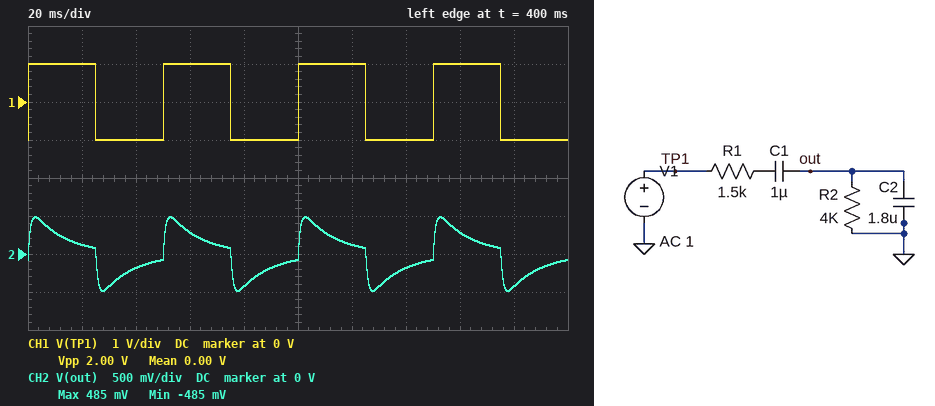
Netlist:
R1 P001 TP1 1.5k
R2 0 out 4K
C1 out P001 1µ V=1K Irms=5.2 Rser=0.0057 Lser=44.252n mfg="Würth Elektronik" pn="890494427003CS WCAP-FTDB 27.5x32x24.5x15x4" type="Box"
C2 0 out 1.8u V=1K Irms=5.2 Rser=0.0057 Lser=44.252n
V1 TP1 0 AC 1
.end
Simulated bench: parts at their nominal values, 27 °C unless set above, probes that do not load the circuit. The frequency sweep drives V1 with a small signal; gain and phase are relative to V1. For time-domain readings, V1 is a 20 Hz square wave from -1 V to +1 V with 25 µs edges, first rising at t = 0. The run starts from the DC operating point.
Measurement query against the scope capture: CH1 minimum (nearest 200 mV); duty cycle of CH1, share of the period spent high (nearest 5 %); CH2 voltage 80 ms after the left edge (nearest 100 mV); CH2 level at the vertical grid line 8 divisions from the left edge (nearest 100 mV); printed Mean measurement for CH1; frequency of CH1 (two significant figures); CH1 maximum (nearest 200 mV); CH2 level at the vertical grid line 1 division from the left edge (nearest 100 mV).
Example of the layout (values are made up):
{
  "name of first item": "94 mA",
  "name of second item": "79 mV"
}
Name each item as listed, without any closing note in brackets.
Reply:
{
  "CH1 minimum": "-1.0 V",
  "duty cycle of CH1, share of the period spent high": "50 %",
  "CH2 voltage 80 ms after the left edge": "-400 mV",
  "CH2 level at the vertical grid line 8 divisions from the left edge": "300 mV",
  "printed Mean measurement for CH1": "0.00 V",
  "frequency of CH1": "20 Hz",
  "CH1 maximum": "1.0 V",
  "CH2 level at the vertical grid line 1 division from the left edge": "100 mV"
}
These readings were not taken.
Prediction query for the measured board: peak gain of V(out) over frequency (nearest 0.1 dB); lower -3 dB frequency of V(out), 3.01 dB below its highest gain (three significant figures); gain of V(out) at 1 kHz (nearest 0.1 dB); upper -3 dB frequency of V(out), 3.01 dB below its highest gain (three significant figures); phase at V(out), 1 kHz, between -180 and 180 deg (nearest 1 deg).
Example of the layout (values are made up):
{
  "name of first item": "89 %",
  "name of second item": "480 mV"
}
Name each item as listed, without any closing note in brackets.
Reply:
{
  "peak gain of V(out) over frequency": "-10.0 dB",
  "lower -3 dB frequency of V(out), 3.01 dB below its highest gain": "11.8 Hz",
  "gain of V(out) at 1 kHz": "-24.7 dB",
  "upper -3 dB frequency of V(out), 3.01 dB below its highest gain": "199 Hz",
  "phase at V(out), 1 kHz, between -180 and 180 deg": "-79 deg"
}
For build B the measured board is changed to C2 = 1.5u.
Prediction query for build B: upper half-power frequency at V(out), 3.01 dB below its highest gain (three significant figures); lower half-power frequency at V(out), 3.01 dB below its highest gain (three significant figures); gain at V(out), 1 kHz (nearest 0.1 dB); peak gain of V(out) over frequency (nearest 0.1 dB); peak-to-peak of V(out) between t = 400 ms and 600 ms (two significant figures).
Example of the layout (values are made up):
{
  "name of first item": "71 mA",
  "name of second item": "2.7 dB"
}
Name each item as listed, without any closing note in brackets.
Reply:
{
  "upper half-power frequency at V(out), 3.01 dB below its highest gain": "216 Hz",
  "lower half-power frequency at V(out), 3.01 dB below its highest gain": "13.0 Hz",
  "gain at V(out), 1 kHz": "-23.2 dB",
  "peak gain of V(out) over frequency": "-9.2 dB",
  "peak-to-peak of V(out) between t = 400 ms and 600 ms": "1.1 V"
}
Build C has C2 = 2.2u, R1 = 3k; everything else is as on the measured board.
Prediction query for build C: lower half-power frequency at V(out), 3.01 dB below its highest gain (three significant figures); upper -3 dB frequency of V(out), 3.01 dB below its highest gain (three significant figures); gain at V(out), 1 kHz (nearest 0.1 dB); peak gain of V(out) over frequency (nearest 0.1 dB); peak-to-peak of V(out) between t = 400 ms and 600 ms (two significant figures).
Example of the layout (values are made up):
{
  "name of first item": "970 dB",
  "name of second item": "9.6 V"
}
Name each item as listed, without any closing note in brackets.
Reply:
{
  "lower half-power frequency at V(out), 3.01 dB below its highest gain": "9.19 Hz",
  "upper -3 dB frequency of V(out), 3.01 dB below its highest gain": "104 Hz",
  "gain at V(out), 1 kHz": "-32.4 dB",
  "peak gain of V(out) over frequency": "-11.9 dB",
  "peak-to-peak of V(out) between t = 400 ms and 600 ms": "700 mV"
}
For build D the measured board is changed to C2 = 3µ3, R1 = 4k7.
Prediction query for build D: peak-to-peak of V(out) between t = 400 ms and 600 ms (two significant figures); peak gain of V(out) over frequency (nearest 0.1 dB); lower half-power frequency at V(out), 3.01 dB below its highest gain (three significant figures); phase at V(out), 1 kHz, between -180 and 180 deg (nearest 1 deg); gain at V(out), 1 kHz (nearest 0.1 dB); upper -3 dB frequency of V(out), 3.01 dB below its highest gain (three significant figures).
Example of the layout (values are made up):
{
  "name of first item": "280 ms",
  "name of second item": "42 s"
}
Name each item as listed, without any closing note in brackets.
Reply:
{
  "peak-to-peak of V(out) between t = 400 ms and 600 ms": "450 mV",
  "peak gain of V(out) over frequency": "-14.8 dB",
  "lower half-power frequency at V(out), 3.01 dB below its highest gain": "6.51 Hz",
  "phase at V(out), 1 kHz, between -180 and 180 deg": "-87 deg",
  "gain at V(out), 1 kHz": "-39.8 dB",
  "upper -3 dB frequency of V(out), 3.01 dB below its highest gain": "62.7 Hz"
}
